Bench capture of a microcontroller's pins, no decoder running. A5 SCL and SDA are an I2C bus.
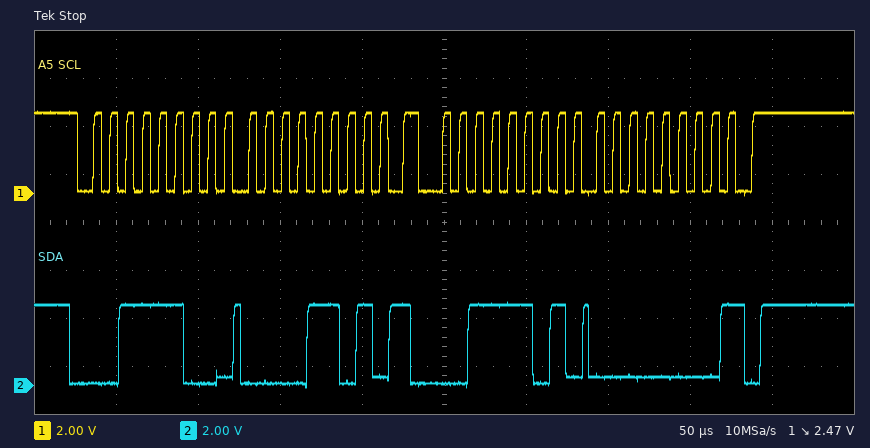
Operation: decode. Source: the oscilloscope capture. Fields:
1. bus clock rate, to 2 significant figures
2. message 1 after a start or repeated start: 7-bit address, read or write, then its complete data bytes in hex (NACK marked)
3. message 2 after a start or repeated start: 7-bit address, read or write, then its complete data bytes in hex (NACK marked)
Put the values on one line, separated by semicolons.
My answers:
100 kHz; 0x1E write: 0D; 0x1E read: 00 NACK
